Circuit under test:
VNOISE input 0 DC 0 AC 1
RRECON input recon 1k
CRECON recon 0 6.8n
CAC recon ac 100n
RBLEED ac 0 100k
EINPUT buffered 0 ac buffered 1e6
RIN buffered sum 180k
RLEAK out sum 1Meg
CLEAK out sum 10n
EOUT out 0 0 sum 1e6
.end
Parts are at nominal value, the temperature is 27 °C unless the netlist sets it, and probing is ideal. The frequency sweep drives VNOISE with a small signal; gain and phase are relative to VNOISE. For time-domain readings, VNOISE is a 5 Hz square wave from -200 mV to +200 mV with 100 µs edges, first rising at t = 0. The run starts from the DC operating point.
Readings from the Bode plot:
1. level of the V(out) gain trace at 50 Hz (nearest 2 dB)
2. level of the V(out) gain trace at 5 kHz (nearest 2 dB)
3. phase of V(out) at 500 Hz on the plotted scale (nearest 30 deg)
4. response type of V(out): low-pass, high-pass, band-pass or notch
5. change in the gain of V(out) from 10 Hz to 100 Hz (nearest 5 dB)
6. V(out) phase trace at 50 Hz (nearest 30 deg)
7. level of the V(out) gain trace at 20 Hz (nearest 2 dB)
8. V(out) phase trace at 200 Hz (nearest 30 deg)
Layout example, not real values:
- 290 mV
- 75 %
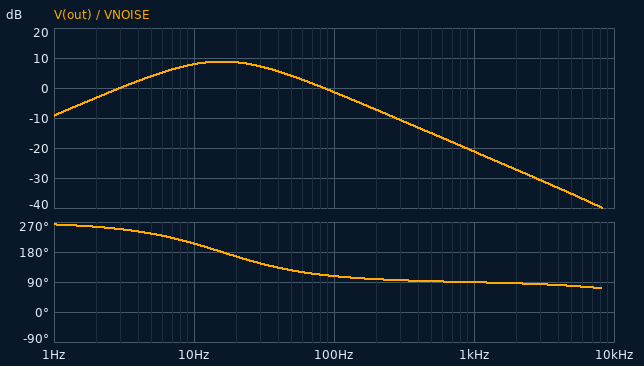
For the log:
- 4 dB
- -36 dB
- 90 deg
- band-pass
- -10 dB
- 120 deg
- 8 dB
- 90 deg
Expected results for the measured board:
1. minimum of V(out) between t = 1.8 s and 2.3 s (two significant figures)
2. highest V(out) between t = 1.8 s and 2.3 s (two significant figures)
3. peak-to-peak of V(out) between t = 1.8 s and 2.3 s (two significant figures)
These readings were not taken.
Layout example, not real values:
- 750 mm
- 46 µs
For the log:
- -810 mV
- 810 mV
- 1.6 V
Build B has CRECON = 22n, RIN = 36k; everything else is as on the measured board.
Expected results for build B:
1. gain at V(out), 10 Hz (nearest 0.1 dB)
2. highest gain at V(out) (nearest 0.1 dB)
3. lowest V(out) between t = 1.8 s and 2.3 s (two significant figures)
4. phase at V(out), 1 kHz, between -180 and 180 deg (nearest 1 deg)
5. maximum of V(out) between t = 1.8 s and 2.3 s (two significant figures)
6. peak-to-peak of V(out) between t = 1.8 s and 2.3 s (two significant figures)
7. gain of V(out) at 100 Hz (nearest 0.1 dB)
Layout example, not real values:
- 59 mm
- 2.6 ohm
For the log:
- 21.9 dB
- 22.8 dB
- -4.1 V
- 84 deg
- 4.1 V
- 8.1 V
- 12.6 dB
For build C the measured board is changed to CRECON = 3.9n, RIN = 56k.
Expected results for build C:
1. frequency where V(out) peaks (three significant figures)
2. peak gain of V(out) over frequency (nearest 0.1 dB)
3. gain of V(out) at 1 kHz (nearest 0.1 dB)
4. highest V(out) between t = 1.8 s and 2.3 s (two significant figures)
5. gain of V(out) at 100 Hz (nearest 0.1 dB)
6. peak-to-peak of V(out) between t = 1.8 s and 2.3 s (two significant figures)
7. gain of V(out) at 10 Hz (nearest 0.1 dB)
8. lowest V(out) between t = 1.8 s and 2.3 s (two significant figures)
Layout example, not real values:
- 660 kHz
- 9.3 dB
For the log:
- 15.8 Hz
- 19.0 dB
- -11.0 dB
- 2.6 V
- 8.8 dB
- 5.2 V
- 18.1 dB
- -2.6 V
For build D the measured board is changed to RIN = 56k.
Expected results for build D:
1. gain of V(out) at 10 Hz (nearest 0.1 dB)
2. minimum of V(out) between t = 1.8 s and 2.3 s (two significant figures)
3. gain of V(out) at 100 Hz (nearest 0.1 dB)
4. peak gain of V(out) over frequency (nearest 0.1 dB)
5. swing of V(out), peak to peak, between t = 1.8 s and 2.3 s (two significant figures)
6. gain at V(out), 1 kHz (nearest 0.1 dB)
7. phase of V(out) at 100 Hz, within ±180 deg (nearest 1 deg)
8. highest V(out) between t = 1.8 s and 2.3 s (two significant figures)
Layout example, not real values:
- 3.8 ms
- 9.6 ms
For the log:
- 18.1 dB
- -2.6 V
- 8.8 dB
- 19.0 dB
- 5.2 V
- -11.0 dB
- 108 deg
- 2.6 V
